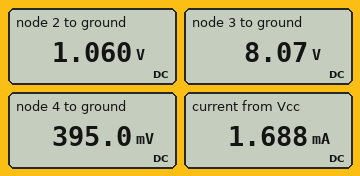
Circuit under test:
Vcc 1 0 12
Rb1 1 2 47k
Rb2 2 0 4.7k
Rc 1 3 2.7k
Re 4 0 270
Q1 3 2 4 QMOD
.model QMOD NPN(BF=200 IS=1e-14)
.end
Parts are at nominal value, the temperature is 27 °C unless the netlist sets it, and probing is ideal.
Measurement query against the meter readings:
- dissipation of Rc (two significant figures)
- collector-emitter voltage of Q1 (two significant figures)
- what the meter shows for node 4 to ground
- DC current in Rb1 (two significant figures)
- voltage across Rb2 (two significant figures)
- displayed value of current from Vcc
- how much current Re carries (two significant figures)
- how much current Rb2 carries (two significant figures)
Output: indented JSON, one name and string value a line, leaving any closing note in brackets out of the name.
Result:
{
  "dissipation of Rc": "5.7 mW",
  "collector-emitter voltage of Q1": "7.7 V",
  "what the meter shows for node 4 to ground": "395.0 mV",
  "DC current in Rb1": "230 µA",
  "voltage across Rb2": "1.1 V",
  "displayed value of current from Vcc": "1.688 mA",
  "how much current Re carries": "1.5 mA",
  "how much current Rb2 carries": "230 µA"
}
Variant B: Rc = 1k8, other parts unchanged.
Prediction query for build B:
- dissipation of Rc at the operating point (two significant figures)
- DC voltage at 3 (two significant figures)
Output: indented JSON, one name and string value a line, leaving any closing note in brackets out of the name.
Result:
{
  "dissipation of Rc at the operating point": "3.8 mW",
  "DC voltage at 3": "9.4 V"
}
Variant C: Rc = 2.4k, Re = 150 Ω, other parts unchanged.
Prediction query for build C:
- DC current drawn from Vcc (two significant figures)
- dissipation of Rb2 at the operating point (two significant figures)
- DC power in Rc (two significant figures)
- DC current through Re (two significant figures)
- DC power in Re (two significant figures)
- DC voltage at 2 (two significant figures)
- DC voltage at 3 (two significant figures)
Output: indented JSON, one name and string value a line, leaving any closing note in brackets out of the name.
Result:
{
  "DC current drawn from Vcc": "2.6 mA",
  "dissipation of Rb2 at the operating point": "230 µW",
  "DC power in Rc": "14 mW",
  "DC current through Re": "2.4 mA",
  "DC power in Re": "870 µW",
  "DC voltage at 2": "1.0 V",
  "DC voltage at 3": "6.2 V"
}
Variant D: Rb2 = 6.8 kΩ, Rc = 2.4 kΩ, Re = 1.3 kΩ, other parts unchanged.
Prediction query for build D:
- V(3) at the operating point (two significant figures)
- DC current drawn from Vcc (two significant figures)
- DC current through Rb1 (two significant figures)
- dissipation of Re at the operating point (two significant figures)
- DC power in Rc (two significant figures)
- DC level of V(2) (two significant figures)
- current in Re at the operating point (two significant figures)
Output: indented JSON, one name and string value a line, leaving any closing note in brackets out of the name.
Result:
{
  "V(3) at the operating point": "10 V",
  "DC current drawn from Vcc": "880 µA",
  "DC current through Rb1": "220 µA",
  "dissipation of Re at the operating point": "560 µW",
  "DC power in Rc": "1.0 mW",
  "DC level of V(2)": "1.5 V",
  "current in Re at the operating point": "660 µA"
}
